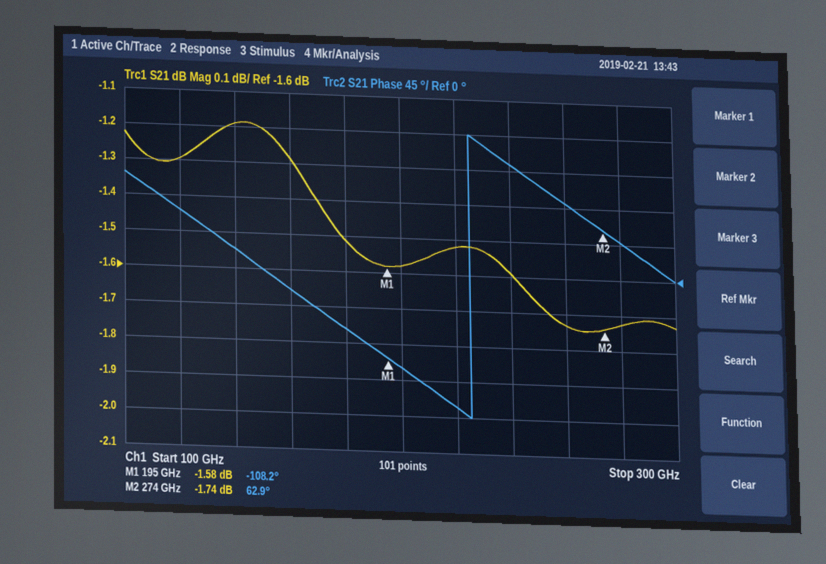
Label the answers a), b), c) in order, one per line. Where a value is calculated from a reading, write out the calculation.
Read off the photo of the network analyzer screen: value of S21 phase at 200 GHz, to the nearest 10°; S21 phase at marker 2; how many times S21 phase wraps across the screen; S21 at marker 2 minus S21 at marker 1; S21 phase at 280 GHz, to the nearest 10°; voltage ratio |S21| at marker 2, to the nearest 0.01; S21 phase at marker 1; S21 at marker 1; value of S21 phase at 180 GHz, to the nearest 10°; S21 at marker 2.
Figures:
a) -120°
b) 62.9°
c) 1
d) -1.74 − (-1.58) = -0.16 dB
e) 50°
f) 10^(-1.74/20) ≈ 0.82
g) -108.2°
h) -1.58 dB
i) -70°
j) -1.74 dB
